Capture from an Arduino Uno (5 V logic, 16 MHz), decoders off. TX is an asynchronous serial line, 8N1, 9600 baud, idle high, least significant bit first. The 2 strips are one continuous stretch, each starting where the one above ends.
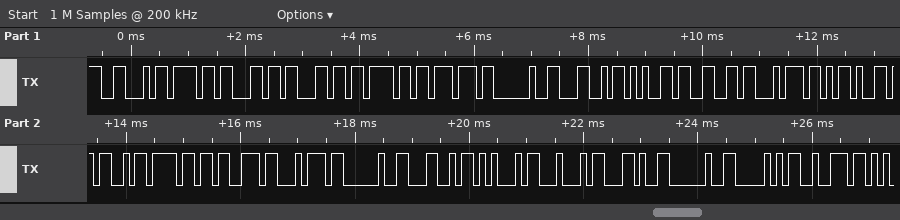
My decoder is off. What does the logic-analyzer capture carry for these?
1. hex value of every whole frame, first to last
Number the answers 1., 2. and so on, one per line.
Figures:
1. 0x46 0x6F 0x6C 0x6C 0x6F 0x77 0x20 0x4C 0x65 0x66 0x74 0x2D 0x4D 0x6F 0x73 0x74 0x20 0x4C 0x45 0x44 0x2C 0x20 0x50 0x72
